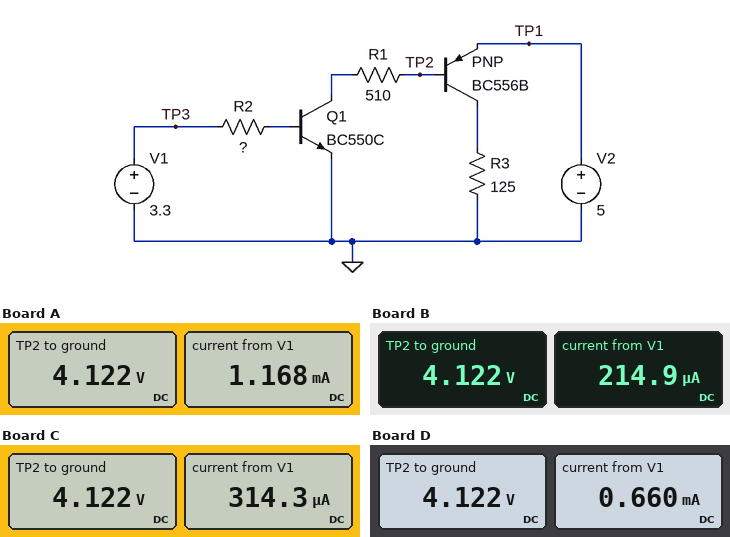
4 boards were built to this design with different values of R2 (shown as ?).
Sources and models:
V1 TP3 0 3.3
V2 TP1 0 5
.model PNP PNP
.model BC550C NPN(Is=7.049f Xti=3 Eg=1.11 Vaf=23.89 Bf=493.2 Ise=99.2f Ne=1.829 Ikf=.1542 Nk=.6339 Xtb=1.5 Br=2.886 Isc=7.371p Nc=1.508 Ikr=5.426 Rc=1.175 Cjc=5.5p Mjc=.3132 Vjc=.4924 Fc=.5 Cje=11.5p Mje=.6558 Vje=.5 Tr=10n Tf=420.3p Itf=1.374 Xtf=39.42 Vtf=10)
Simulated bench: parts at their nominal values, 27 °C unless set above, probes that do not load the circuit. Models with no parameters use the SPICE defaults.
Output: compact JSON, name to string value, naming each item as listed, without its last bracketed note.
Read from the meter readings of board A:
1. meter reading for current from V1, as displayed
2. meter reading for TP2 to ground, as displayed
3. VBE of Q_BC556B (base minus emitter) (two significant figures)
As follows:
{"meter reading for current from V1, as displayed": "1.168 mA", "meter reading for TP2 to ground, as displayed": "4.122 V", "VBE of Q_BC556B (base minus emitter)": "-880 mV"}
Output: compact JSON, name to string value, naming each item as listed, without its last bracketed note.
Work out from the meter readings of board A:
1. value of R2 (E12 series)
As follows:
{"value of R2": "2.2 kΩ"}
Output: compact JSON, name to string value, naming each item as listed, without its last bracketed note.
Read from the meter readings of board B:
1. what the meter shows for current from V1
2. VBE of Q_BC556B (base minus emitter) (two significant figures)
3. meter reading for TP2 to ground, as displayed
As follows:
{"what the meter shows for current from V1": "214.9 µA", "VBE of Q_BC556B (base minus emitter)": "-880 mV", "meter reading for TP2 to ground, as displayed": "4.122 V"}
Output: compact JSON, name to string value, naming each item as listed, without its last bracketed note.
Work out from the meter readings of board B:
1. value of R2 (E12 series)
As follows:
{"value of R2": "12 kΩ"}
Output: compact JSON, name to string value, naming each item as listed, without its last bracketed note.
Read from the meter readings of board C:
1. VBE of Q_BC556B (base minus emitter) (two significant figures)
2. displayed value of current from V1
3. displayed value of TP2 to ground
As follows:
{"VBE of Q_BC556B (base minus emitter)": "-880 mV", "displayed value of current from V1": "314.3 µA", "displayed value of TP2 to ground": "4.122 V"}
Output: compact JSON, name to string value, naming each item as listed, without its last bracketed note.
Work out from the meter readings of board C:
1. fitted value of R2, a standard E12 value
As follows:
{"fitted value of R2, a standard E12 value": "8.2 kΩ"}
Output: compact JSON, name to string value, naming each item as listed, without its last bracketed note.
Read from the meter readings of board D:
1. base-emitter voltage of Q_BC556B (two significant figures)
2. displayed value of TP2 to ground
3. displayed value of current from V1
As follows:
{"base-emitter voltage of Q_BC556B": "-880 mV", "displayed value of TP2 to ground": "4.122 V", "displayed value of current from V1": "0.660 mA"}
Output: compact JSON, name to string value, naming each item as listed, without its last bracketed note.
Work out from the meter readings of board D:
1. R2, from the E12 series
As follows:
{"R2, from the E12 series": "3.9 kΩ"}
